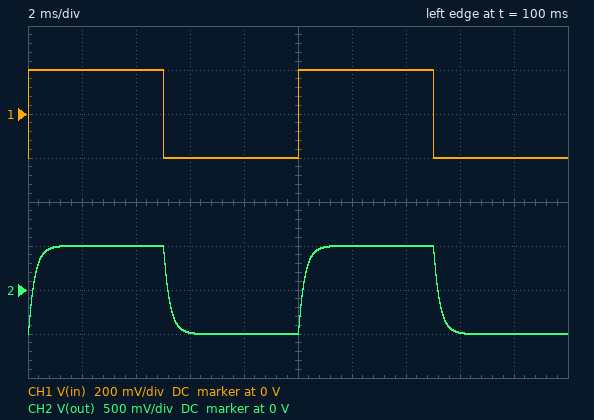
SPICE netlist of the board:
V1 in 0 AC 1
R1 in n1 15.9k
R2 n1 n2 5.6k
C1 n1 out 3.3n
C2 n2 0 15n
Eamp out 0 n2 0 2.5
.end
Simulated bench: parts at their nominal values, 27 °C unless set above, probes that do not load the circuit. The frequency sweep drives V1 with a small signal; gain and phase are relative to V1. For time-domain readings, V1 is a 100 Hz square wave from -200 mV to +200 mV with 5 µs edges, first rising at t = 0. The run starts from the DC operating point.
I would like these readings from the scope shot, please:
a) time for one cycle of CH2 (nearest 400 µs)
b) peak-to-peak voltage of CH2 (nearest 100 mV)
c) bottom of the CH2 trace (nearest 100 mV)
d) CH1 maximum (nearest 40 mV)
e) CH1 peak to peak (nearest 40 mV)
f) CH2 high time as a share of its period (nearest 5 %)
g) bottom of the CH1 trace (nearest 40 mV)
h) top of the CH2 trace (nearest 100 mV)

10.0 ms
1.0 V
-500 mV
200 mV
400 mV
50 %
-200 mV
500 mV
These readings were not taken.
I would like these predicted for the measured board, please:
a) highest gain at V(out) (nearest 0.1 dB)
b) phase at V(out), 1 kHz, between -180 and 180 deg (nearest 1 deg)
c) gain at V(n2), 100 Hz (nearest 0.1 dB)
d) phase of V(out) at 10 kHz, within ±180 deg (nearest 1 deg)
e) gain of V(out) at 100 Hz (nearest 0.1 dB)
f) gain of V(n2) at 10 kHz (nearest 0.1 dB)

8.0 dB
-62 deg
-0.1 dB
-137 deg
7.9 dB
-27.0 dB
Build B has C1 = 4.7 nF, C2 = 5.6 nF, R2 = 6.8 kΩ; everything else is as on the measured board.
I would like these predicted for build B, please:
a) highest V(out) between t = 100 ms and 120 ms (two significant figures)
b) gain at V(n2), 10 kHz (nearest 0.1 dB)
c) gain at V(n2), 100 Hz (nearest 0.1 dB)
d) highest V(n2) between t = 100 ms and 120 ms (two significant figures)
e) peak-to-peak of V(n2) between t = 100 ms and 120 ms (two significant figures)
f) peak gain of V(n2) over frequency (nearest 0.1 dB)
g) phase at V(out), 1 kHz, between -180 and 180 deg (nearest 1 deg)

1.1 V
-20.2 dB
0 dB
460 mV
910 mV
11.1 dB
-6 deg
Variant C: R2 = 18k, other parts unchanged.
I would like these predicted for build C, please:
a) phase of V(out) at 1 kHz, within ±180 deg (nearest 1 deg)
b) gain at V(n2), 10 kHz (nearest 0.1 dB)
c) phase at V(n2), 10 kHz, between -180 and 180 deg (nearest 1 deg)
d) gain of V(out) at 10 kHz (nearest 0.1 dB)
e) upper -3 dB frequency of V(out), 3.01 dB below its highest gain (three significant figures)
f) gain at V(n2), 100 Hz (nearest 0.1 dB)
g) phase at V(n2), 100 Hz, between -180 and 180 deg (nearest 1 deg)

-81 deg
-35.7 dB
-154 deg
-27.8 dB
401 Hz
-0.3 dB
-15 deg
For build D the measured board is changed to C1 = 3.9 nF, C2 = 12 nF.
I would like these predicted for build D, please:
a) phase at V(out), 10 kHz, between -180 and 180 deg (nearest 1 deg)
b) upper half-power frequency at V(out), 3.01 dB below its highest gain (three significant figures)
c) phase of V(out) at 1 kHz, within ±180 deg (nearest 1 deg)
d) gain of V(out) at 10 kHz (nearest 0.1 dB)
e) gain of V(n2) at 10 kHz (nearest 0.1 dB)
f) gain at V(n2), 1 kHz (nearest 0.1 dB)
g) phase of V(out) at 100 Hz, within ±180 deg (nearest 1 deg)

-146 deg
1.13 kHz
-51 deg
-17.4 dB
-25.4 dB
-2.5 dB
-6 deg
